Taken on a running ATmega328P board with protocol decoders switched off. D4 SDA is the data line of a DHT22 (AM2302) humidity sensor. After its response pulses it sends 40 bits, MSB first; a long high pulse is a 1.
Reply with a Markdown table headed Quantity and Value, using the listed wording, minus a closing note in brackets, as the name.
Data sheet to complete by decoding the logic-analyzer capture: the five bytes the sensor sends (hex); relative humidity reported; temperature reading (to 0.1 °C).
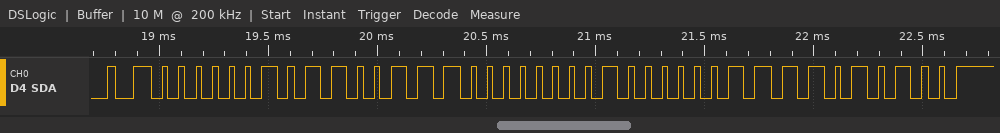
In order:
| Quantity | Value |
|---|---|
| the five bytes the sensor sends | 02 CE 01 03 D4 |
| relative humidity reported | 71.8 % |
| temperature reading | 25.9 °C |
